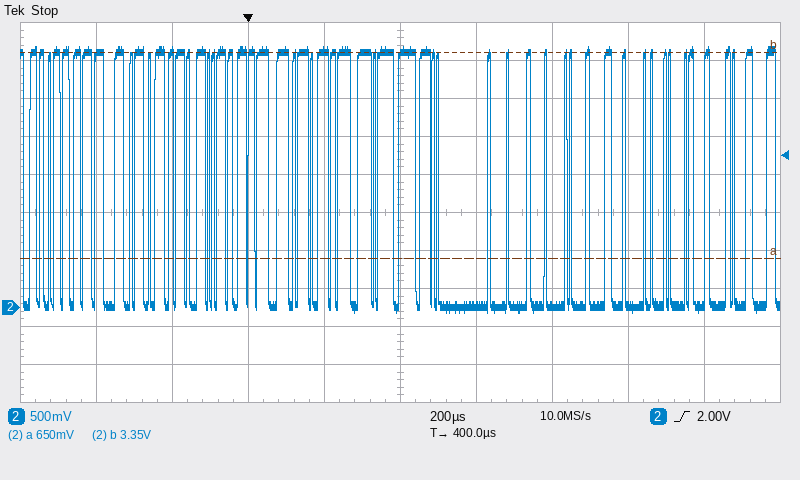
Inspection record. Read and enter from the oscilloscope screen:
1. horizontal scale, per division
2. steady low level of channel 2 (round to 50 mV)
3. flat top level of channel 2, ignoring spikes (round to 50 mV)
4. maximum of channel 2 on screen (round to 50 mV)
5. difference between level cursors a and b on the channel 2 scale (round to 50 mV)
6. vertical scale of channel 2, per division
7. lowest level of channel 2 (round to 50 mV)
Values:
200 µs
0 mV
3.35 V
3.45 V
2.70 V
500 mV
-100 mV
